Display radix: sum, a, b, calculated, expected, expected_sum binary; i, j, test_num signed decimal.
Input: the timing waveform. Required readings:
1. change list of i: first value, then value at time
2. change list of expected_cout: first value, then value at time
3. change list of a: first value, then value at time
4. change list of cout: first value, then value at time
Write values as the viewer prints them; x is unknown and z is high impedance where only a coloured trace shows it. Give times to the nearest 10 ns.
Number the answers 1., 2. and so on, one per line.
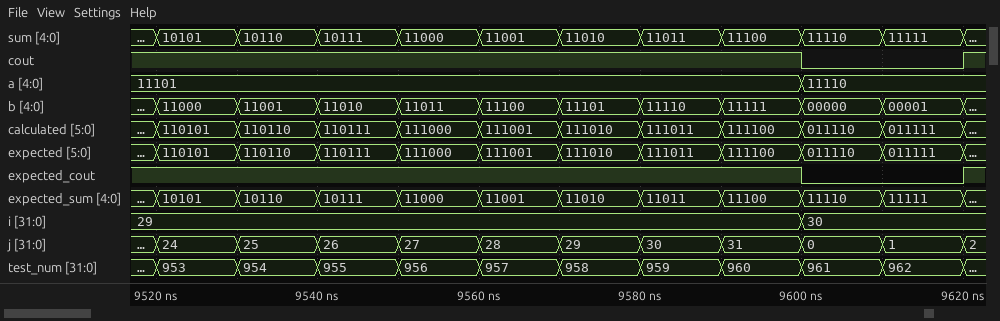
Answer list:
1. 29, 30 at 9600 ns
2. 1, 0 at 9600 ns, 1 at 9620 ns
3. 11101, 11110 at 9600 ns
4. 1, 0 at 9600 ns, 1 at 9620 ns
